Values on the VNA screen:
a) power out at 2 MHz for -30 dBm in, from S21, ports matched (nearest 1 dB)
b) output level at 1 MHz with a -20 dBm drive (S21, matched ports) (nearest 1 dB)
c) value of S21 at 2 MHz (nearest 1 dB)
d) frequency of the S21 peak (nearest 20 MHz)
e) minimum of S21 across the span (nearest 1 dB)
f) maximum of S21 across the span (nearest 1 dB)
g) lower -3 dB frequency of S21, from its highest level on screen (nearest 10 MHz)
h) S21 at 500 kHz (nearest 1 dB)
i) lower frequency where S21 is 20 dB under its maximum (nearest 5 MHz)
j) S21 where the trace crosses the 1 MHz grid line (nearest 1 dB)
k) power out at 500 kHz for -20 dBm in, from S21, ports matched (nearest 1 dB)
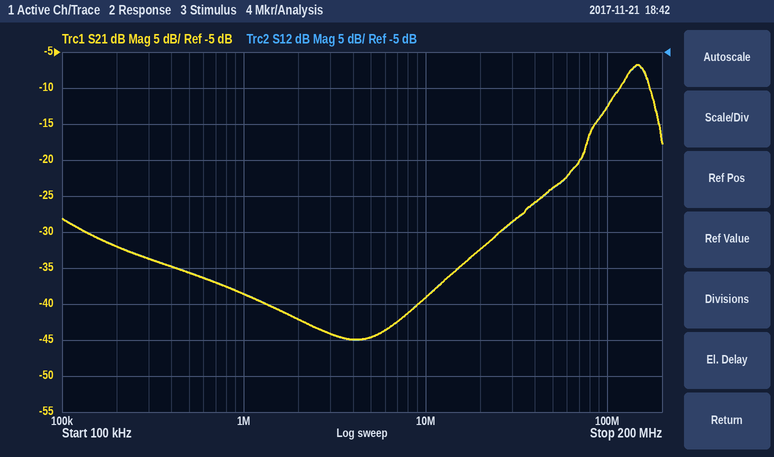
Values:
-72 dBm
-59 dBm
-42 dB
140 MHz
-45 dB
-7 dB
120 MHz
-36 dB
35 MHz
-39 dB
-56 dBm
